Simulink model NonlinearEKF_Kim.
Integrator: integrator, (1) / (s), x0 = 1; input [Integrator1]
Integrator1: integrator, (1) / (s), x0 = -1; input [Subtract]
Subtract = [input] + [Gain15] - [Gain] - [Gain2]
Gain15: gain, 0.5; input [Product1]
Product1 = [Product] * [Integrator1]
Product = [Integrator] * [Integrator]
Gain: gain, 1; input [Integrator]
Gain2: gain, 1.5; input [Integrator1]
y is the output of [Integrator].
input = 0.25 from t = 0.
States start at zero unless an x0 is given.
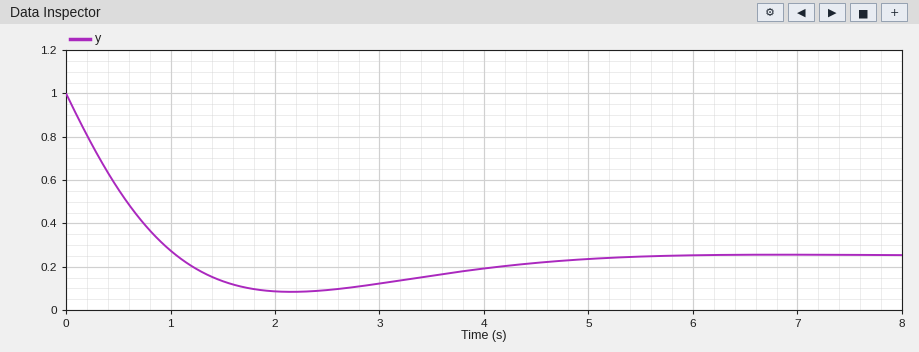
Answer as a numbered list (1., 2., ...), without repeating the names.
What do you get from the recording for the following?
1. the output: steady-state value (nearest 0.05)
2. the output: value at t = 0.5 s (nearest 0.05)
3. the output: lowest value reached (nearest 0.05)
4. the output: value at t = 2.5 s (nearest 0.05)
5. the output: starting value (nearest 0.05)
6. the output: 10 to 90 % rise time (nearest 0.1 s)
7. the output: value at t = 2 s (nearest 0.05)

1. 0.25
2. 0.55
3. 0.10
4. 0.10
5. 1.00
6. 0.8 s
7. 0.10
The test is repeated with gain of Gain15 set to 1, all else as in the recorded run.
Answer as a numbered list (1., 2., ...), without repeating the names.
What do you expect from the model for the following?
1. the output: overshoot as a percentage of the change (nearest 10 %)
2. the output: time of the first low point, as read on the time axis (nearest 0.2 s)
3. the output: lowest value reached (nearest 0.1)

1. 30 %
2. 2.0 s
3. 0.0
